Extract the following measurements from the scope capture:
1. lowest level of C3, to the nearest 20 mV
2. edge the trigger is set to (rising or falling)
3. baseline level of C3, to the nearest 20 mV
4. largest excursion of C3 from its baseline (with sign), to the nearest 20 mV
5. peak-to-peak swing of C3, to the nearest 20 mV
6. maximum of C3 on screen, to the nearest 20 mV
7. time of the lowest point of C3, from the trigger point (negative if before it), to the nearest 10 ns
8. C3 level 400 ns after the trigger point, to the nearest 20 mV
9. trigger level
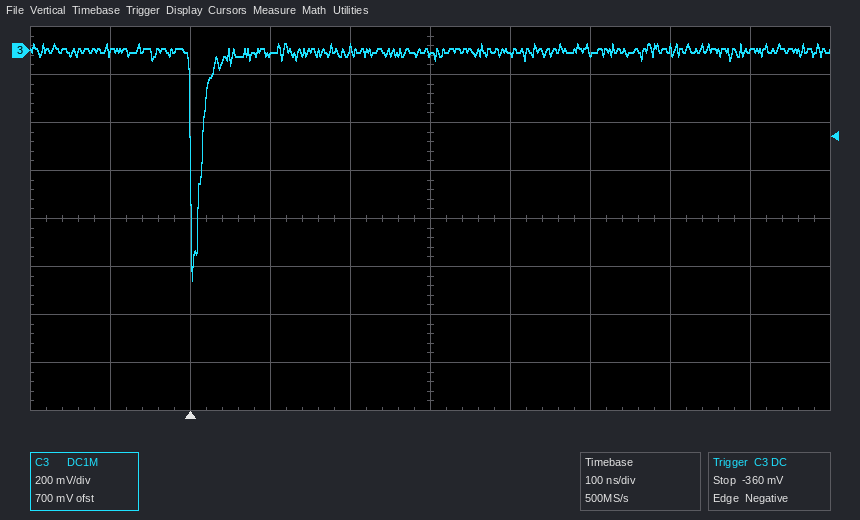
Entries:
-960 mV
falling
0 mV
-960 mV
980 mV
20 mV
0 ns
0 mV
-360 mV
